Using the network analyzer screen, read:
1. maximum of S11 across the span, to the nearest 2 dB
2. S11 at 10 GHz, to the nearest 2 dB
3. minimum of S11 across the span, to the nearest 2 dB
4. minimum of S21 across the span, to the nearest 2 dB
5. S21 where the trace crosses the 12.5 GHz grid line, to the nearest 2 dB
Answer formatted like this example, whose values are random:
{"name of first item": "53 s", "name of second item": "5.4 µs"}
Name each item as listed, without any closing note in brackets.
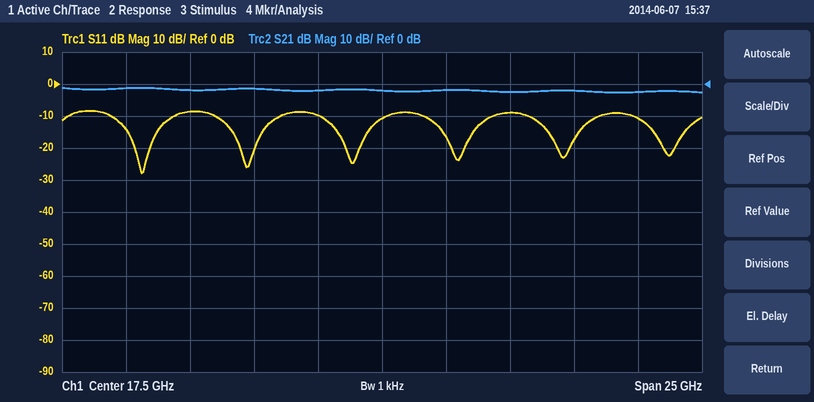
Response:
{"maximum of S11 across the span, to the nearest 2 dB": "-8 dB", "S11 at 10 GHz, to the nearest 2 dB": "-8 dB", "minimum of S11 across the span, to the nearest 2 dB": "-28 dB", "minimum of S21 across the span, to the nearest 2 dB": "-2 dB", "S21 where the trace crosses the 12.5 GHz grid line, to the nearest 2 dB": "-2 dB"}
